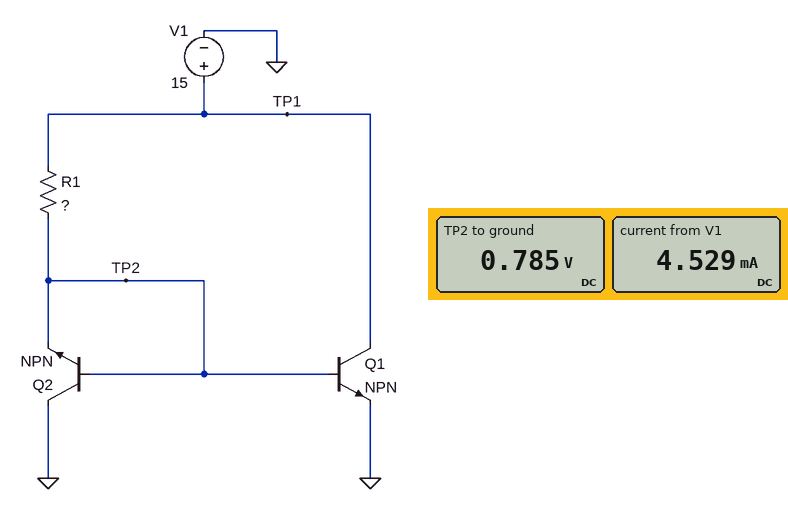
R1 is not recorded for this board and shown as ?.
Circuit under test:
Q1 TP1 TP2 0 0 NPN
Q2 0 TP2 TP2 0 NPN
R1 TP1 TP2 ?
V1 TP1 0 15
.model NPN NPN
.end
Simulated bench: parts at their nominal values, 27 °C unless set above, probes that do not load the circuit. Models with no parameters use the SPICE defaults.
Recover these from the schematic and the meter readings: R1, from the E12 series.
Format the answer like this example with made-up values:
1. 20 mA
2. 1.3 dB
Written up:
1. 4.7 kΩ
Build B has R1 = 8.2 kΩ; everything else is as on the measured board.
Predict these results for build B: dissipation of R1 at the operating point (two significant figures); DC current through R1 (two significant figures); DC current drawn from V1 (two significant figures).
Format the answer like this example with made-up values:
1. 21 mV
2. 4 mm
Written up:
1. 25 mW
2. 1.7 mA
3. 2.6 mA
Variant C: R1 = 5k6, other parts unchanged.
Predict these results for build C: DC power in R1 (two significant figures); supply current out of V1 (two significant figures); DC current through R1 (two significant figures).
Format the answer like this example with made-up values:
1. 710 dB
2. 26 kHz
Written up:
1. 36 mW
2. 3.8 mA
3. 2.5 mA
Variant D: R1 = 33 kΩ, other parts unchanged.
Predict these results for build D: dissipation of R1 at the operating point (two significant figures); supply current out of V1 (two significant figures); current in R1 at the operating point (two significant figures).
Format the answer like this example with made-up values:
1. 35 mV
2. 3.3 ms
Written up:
1. 6.2 mW
2. 650 µA
3. 430 µA
